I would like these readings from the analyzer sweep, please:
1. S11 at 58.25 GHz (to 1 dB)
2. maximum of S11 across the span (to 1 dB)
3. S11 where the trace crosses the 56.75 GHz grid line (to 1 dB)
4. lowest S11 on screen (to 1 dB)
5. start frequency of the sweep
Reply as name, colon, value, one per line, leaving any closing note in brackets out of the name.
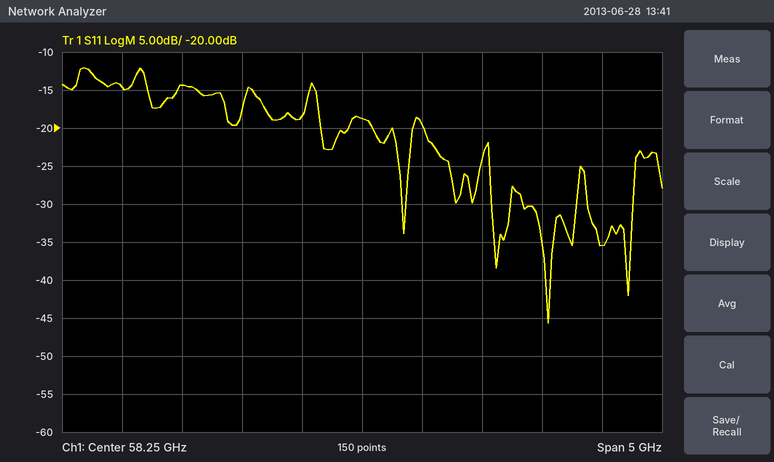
S11 at 58.25 GHz: -19 dB
maximum of S11 across the span: -12 dB
S11 where the trace crosses the 56.75 GHz grid line: -14 dB
lowest S11 on screen: -46 dB
start frequency of the sweep: 55.75 GHz
